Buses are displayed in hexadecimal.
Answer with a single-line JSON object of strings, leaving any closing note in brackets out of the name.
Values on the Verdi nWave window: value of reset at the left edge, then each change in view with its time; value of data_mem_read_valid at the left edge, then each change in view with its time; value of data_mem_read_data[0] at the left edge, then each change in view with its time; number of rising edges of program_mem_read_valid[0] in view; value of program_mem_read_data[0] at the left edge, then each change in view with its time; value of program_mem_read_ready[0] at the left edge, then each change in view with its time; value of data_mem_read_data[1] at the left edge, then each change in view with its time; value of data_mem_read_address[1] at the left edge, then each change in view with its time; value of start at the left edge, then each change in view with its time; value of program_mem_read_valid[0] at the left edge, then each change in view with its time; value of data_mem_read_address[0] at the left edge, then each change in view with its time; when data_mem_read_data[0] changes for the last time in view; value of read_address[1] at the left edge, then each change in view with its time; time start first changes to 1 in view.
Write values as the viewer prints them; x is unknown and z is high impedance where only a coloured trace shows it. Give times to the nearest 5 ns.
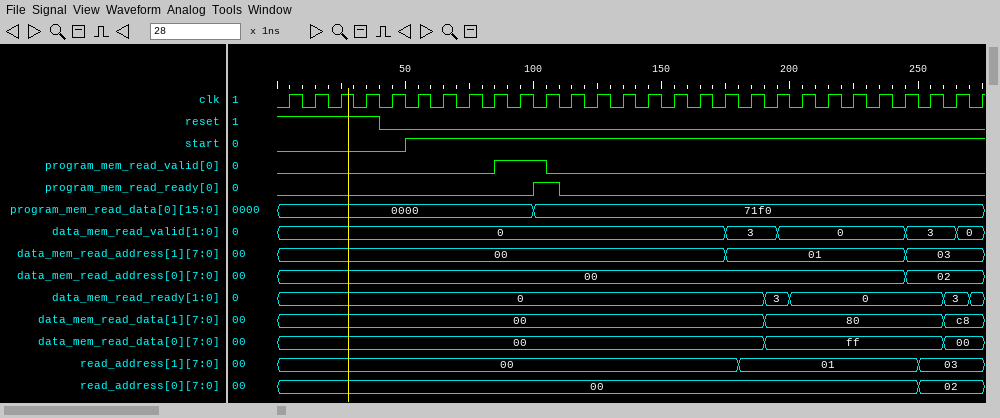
{"value of reset at the left edge, then each change in view with its time": "1, 0 at 40 ns", "value of data_mem_read_valid at the left edge, then each change in view with its time": "0, 3 at 175 ns, 0 at 195 ns, 3 at 245 ns, 0 at 265 ns", "value of data_mem_read_data[0] at the left edge, then each change in view with its time": "00, ff at 190 ns, 00 at 260 ns", "number of rising edges of program_mem_read_valid[0] in view": "1", "value of program_mem_read_data[0] at the left edge, then each change in view with its time": "0000, 71f0 at 100 ns", "value of program_mem_read_ready[0] at the left edge, then each change in view with its time": "0, 1 at 100 ns, 0 at 110 ns", "value of data_mem_read_data[1] at the left edge, then each change in view with its time": "00, 80 at 190 ns, c8 at 260 ns", "value of data_mem_read_address[1] at the left edge, then each change in view with its time": "00, 01 at 175 ns, 03 at 245 ns", "value of start at the left edge, then each change in view with its time": "0, 1 at 50 ns", "value of program_mem_read_valid[0] at the left edge, then each change in view with its time": "0, 1 at 85 ns, 0 at 105 ns", "value of data_mem_read_address[0] at the left edge, then each change in view with its time": "00, 02 at 245 ns", "when data_mem_read_data[0] changes for the last time in view": "260 ns", "value of read_address[1] at the left edge, then each change in view with its time": "00, 01 at 180 ns, 03 at 250 ns", "time start first changes to 1 in view": "50 ns"}
